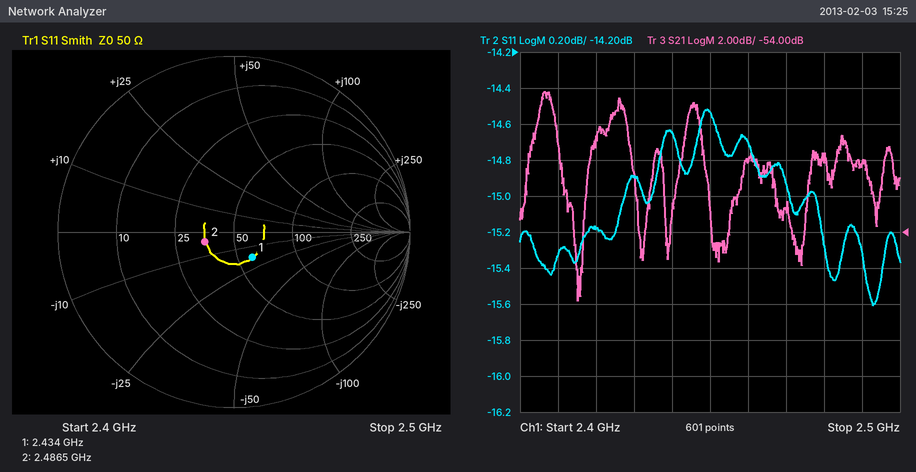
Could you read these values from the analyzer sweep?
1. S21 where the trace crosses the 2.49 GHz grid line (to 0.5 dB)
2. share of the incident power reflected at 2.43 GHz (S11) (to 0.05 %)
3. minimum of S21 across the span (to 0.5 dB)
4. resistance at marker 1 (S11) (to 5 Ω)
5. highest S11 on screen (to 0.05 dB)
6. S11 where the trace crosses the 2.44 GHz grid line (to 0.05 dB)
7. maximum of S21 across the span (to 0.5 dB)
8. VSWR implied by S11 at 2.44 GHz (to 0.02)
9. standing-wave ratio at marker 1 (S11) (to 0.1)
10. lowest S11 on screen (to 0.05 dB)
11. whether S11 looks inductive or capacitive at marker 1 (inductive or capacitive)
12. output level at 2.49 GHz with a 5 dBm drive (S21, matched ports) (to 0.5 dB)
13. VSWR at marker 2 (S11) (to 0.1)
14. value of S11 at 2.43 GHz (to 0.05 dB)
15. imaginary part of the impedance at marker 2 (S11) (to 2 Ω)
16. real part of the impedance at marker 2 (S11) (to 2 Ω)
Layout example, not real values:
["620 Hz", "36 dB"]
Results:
["-50.0 dB", "3.25 %", "-58.0 dB", "60 Ω", "-14.50 dB", "-14.65 dB", "-46.0 dB", "1.46", "1.4", "-15.60 dB", "capacitive", "-45.0 dBm", "1.4", "-14.90 dB", "-4 Ω", "36 Ω"]
